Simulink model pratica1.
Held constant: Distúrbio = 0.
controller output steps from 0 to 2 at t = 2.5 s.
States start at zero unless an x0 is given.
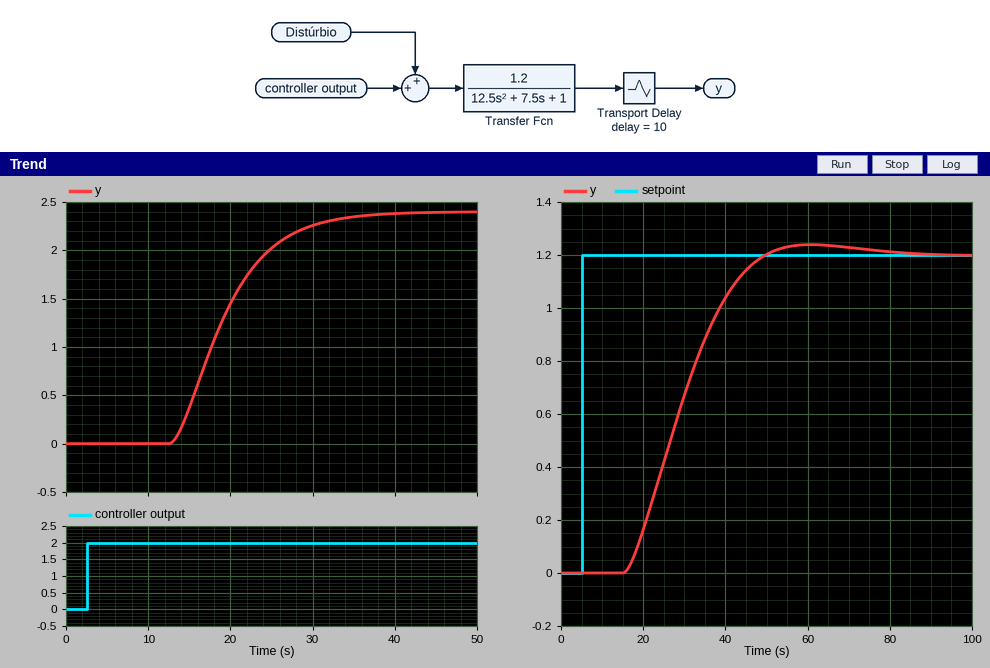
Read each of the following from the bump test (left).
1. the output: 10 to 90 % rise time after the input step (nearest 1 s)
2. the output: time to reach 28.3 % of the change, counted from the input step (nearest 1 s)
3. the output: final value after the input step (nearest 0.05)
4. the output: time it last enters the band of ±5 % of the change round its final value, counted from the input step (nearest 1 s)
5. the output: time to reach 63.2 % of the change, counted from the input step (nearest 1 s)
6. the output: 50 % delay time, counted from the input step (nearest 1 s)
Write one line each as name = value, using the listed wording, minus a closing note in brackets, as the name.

the output: 10 to 90 % rise time after the input step = 13 s
the output: time to reach 28.3 % of the change, counted from the input step = 14 s
the output: final value after the input step = 2.40
the output: time it last enters the band of ±5 % of the change round its final value, counted from the input step = 28 s
the output: time to reach 63.2 % of the change, counted from the input step = 18 s
the output: 50 % delay time, counted from the input step = 16 s
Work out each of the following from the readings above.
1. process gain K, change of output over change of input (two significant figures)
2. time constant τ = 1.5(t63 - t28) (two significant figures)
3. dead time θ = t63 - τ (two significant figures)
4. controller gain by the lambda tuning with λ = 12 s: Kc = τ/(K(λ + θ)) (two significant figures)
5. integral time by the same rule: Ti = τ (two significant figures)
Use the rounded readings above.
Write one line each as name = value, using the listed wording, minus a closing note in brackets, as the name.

process gain K, change of output over change of input = 1.2
time constant τ = 1.5(t63 - t28) = 6.0 s
dead time θ = t63 - τ = 12 s
controller gain by the lambda tuning with λ = 12 s: Kc = τ/(K(λ + θ)) = 0.21
integral time by the same rule: Ti = τ = 6.0 s
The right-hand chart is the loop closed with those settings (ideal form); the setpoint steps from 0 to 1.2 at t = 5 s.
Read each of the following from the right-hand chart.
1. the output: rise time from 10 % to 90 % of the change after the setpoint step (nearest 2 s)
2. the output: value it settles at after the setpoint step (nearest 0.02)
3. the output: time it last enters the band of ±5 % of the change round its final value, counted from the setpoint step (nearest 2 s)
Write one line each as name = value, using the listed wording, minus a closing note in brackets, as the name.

the output: rise time from 10 % to 90 % of the change after the setpoint step = 22 s
the output: value it settles at after the setpoint step = 1.20
the output: time it last enters the band of ±5 % of the change round its final value, counted from the setpoint step = 40 s
